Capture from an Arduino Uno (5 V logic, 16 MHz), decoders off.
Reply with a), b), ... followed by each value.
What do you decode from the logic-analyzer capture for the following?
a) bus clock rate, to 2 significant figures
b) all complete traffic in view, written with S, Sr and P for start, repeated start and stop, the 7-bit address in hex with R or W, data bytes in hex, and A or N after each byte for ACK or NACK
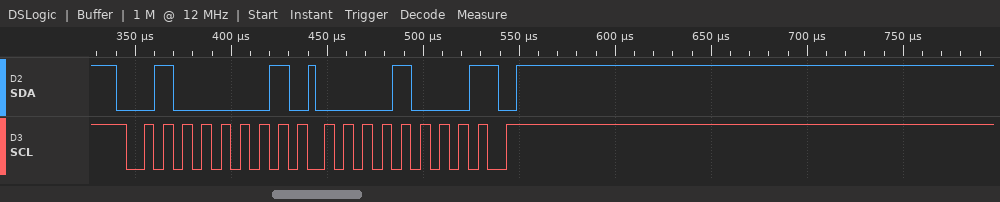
a) 100 kHz
b) S 20R A 08 N P
